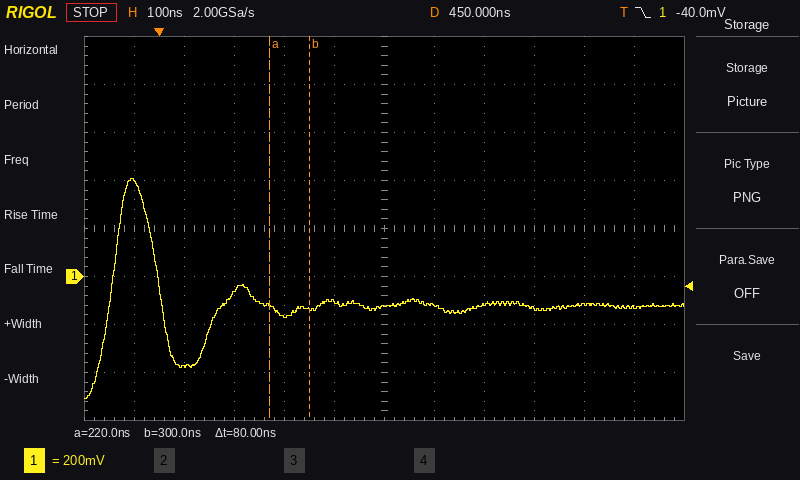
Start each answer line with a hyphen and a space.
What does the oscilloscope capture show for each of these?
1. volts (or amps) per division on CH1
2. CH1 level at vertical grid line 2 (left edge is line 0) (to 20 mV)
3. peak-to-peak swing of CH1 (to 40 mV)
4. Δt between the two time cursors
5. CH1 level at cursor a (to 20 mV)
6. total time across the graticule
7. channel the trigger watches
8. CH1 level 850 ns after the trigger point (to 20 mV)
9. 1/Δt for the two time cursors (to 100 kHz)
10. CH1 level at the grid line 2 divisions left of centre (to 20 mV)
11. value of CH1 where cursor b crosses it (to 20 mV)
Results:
- 200 mV
- -380 mV
- 920 mV
- 80 ns
- -120 mV
- 1.2 µs
- CH1
- -120 mV
- 12.5 MHz
- -160 mV
- -140 mV
